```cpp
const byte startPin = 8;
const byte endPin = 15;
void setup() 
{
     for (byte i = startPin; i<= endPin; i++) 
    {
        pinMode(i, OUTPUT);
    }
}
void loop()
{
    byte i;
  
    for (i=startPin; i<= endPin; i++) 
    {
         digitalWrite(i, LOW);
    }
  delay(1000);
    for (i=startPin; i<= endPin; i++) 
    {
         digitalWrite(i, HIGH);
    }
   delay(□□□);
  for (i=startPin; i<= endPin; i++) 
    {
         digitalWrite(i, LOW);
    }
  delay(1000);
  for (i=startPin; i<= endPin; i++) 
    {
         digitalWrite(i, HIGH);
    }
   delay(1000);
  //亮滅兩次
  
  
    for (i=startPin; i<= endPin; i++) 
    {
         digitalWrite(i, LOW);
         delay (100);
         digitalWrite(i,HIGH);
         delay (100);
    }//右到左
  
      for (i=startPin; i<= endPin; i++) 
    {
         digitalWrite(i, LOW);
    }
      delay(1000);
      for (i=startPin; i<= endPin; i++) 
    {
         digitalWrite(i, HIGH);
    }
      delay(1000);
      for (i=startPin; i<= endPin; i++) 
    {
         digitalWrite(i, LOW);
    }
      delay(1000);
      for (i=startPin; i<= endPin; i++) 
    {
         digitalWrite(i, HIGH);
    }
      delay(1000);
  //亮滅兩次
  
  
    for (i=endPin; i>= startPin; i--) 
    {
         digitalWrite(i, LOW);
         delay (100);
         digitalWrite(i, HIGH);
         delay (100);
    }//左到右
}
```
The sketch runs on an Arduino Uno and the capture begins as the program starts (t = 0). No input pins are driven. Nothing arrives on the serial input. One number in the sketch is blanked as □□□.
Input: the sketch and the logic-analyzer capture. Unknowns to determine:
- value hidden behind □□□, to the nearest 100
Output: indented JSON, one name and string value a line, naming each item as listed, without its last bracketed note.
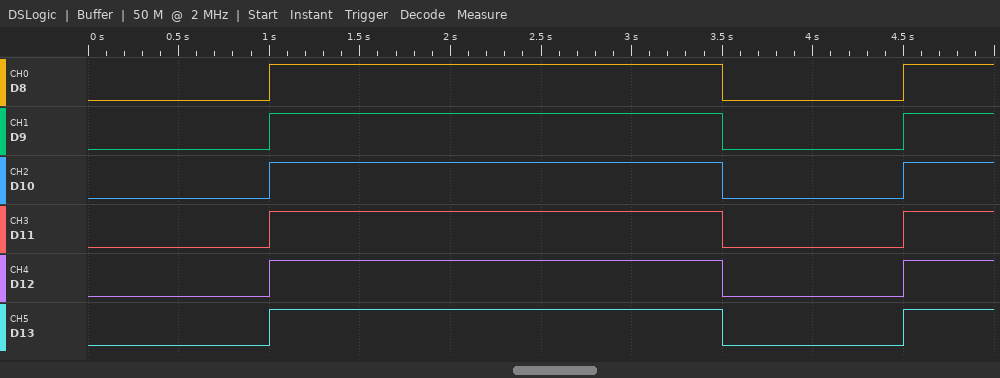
{
  "value hidden behind □□□, to the nearest 100": "2500"
}
